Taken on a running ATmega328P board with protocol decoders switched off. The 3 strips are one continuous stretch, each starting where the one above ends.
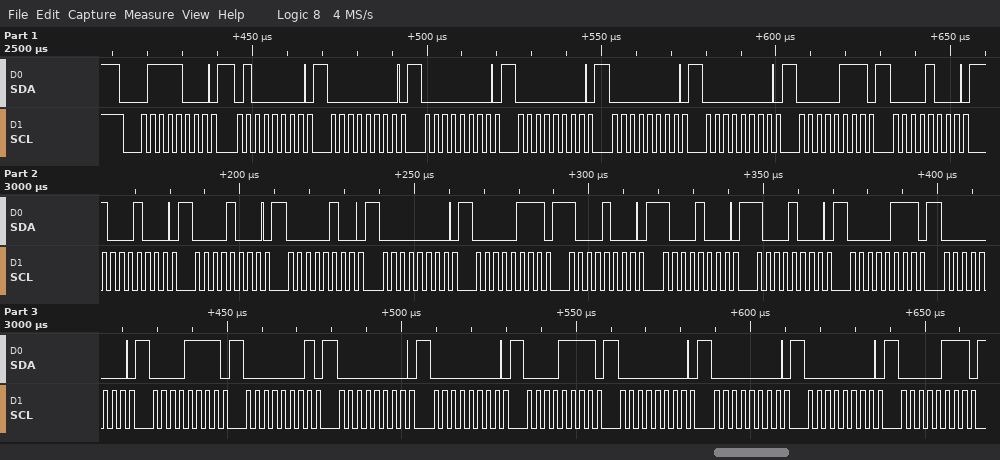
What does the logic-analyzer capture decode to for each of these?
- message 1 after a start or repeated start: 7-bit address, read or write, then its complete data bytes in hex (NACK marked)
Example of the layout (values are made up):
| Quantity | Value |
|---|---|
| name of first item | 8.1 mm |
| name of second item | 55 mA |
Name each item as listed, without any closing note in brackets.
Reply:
| Quantity | Value |
|---|---|
| message 1 after a start or repeated start: 7-bit address, read or write, then its complete data bytes in hex | 0x3C write: 40 00 00 00 00 00 07 08 88 08 04 00 07 88 88 88 07 00 0F 01 00 00 0F 00 00 00 07 |
